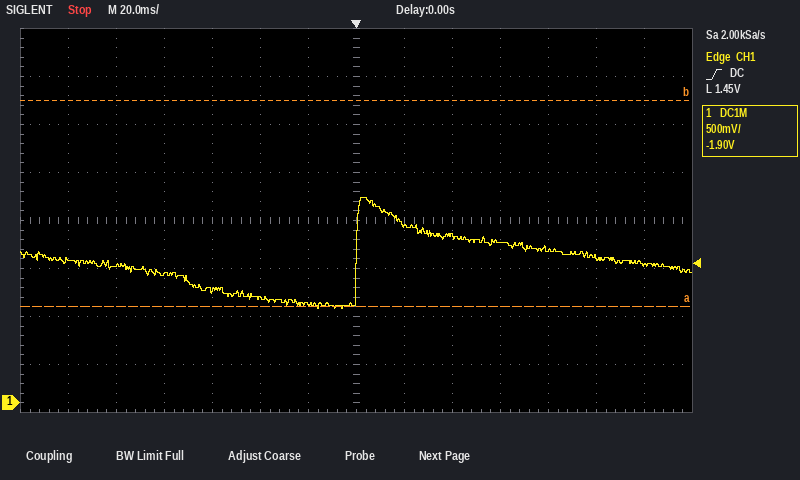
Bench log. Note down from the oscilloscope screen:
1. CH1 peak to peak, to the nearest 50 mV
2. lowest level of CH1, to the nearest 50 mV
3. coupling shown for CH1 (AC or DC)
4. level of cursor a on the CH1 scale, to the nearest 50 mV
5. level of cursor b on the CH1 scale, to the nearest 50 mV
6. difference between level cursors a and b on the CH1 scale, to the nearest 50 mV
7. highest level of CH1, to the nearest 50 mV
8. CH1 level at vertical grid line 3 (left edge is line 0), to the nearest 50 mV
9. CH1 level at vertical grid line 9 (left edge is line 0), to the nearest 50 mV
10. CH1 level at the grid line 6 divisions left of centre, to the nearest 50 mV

1.15 V
1.00 V
DC
1.00 V
3.15 V
2.15 V
2.15 V
1.35 V
1.75 V
1.50 V
